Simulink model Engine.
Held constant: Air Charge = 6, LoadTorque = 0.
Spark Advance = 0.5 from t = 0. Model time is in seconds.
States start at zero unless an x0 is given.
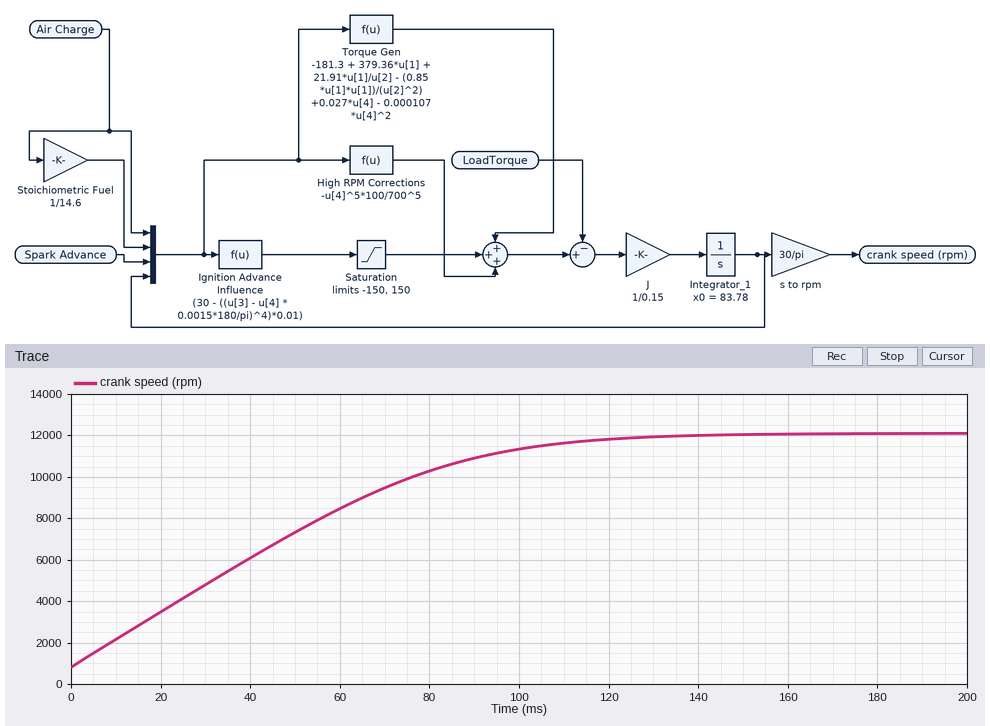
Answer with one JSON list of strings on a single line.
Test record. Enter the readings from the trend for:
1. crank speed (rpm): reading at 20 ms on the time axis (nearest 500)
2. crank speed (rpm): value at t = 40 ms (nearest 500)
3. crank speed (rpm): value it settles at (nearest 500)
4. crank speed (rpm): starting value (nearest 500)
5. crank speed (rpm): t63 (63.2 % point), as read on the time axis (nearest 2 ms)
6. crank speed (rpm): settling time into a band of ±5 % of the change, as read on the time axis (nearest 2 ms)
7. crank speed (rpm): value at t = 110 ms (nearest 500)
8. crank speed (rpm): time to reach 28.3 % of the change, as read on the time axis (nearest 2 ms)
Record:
["3500", "6000", "12000", "1000", "56 ms", "106 ms", "11500", "24 ms"]
